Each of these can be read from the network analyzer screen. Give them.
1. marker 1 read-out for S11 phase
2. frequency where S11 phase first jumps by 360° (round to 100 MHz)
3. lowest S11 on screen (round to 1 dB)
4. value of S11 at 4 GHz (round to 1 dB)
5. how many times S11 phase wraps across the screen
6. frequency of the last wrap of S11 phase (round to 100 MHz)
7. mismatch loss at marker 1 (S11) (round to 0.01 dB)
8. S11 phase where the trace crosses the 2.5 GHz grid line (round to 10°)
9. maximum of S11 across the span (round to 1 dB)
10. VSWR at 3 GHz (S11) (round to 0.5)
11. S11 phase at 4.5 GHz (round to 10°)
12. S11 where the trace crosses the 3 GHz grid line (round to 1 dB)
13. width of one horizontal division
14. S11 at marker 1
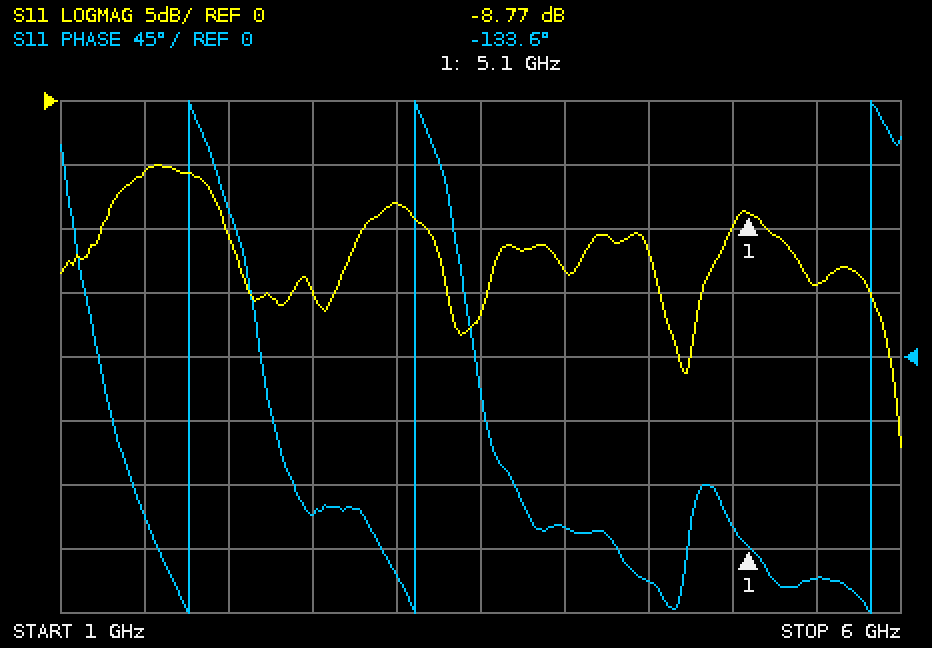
-133.6°
1.8 GHz
-27 dB
-13 dB
3
5.8 GHz
0.62 dB
-110°
-5 dB
2.5
-160°
-8 dB
500 MHz
-8.77 dB
